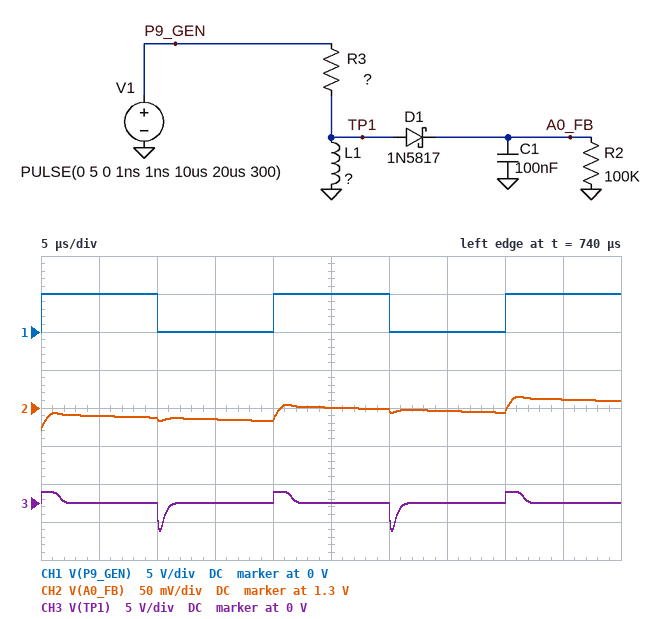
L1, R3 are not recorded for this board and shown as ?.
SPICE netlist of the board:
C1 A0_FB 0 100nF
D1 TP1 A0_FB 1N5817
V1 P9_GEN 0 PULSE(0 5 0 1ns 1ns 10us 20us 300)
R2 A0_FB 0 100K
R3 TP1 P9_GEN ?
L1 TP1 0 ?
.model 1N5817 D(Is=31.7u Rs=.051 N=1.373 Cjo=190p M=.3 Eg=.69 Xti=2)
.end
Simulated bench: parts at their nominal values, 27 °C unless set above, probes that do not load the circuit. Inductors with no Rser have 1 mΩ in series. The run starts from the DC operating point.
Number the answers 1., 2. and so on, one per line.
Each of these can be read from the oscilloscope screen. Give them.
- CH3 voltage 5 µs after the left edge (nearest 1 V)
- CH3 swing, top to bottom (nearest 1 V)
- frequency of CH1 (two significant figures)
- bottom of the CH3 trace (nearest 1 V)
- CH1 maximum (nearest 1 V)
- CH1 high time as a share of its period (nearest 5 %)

1. 0 V
2. 5 V
3. 50 kHz
4. -4 V
5. 5 V
6. 50 %
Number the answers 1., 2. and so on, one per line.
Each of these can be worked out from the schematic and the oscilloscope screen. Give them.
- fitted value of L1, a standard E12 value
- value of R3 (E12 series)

1. 470 µH
2. 1 kΩ
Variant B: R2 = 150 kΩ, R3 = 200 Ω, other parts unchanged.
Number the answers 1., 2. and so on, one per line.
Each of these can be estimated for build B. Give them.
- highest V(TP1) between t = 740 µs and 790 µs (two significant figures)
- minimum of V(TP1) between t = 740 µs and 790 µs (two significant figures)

1. 3.7 V
2. -4.8 V
